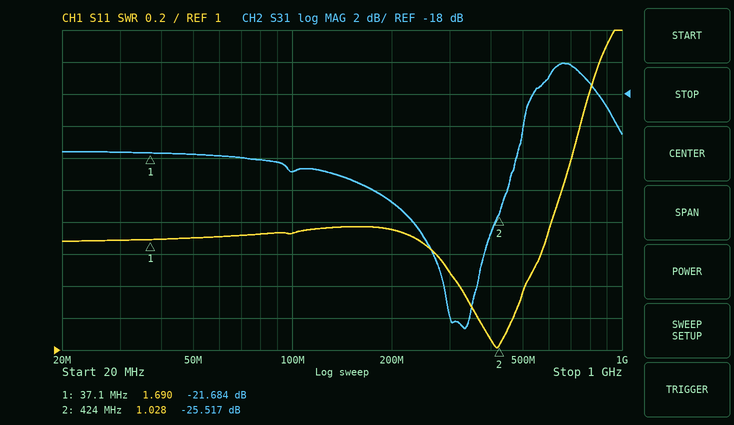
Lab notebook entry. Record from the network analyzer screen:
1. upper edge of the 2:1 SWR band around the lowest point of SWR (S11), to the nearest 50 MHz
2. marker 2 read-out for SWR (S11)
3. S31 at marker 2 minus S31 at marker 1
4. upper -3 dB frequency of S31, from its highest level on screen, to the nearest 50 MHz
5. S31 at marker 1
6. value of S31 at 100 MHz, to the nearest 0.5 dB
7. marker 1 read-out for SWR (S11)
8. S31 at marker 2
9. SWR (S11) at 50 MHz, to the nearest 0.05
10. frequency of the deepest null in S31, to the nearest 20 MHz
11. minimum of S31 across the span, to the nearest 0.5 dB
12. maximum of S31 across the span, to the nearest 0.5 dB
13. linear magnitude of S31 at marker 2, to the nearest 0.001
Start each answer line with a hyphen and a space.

- 650 MHz
- 1.028
- -3.833 dB
- 900 MHz
- -21.684 dB
- -23.0 dB
- 1.690
- -25.517 dB
- 1.70
- 340 MHz
- -32.5 dB
- -16.0 dB
- 0.053
